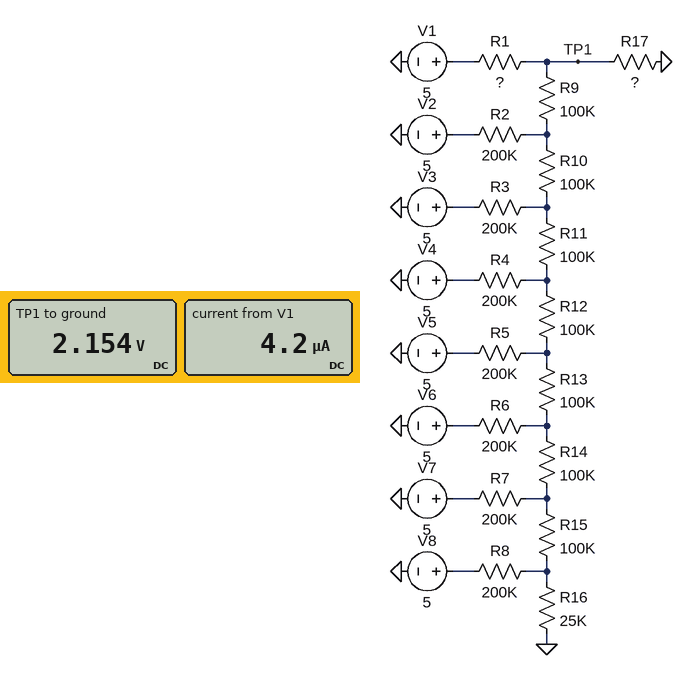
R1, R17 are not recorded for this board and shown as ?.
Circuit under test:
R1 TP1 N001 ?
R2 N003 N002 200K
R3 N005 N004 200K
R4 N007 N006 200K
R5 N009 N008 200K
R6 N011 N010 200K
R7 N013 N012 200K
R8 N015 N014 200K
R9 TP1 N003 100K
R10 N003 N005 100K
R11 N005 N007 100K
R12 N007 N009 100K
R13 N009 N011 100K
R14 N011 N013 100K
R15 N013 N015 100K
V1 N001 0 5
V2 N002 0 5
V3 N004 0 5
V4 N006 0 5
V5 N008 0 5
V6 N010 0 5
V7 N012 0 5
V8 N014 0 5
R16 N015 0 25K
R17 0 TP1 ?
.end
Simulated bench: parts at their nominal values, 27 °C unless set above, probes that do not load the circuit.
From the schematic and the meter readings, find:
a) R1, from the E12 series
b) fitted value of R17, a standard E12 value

680 kΩ
120 kΩ
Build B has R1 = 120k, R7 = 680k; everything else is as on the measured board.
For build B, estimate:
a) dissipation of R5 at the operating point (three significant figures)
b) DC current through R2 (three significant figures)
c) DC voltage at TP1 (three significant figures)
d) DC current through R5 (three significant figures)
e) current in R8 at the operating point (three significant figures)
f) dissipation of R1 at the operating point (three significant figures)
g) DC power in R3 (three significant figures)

2.74 µW
5.17 µA
3.05 V
3.70 µA
20.5 µA
31.7 µW
2.00 µW
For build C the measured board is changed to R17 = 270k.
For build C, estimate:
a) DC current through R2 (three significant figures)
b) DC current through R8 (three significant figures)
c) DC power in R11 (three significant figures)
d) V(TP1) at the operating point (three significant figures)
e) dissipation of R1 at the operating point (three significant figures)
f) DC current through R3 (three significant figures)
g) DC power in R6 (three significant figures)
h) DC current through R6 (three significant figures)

4.90 µA
20.0 µA
110 nW
3.13 V
5.12 µW
2.92 µA
5.56 µW
5.27 µA
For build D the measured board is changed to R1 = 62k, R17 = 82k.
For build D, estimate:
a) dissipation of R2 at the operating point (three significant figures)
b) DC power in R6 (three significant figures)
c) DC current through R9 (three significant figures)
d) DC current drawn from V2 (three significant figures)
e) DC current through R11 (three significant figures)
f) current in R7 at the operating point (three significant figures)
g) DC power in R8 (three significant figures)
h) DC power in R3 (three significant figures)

4.69 µW
5.56 µW
8.75 µA
4.84 µA
1.02 µA
10.1 µA
80.2 µW
1.67 µW
